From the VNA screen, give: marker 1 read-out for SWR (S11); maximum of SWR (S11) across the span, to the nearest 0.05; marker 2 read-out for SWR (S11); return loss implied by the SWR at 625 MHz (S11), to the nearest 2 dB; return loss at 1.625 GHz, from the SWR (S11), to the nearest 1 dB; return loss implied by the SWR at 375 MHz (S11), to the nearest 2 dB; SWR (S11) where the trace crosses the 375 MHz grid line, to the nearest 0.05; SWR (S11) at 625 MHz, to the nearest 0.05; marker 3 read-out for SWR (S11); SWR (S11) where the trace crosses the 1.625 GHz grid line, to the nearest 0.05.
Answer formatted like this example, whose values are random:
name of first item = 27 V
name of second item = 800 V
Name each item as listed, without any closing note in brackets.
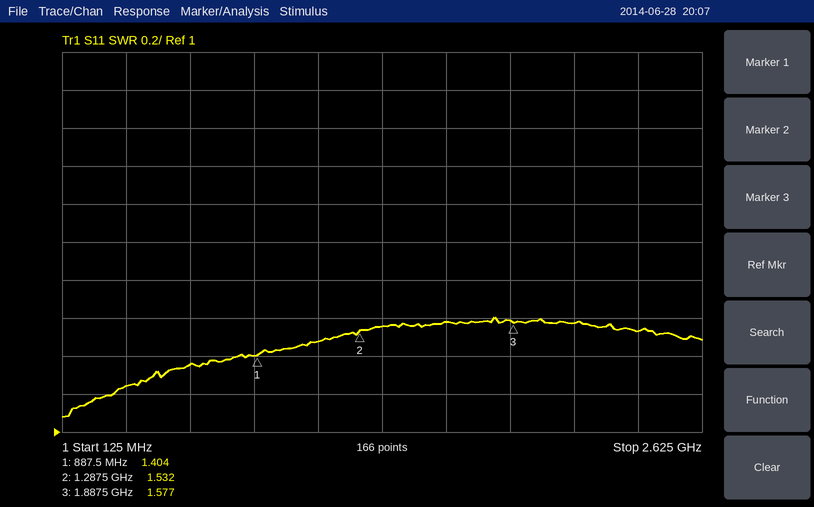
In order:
marker 1 read-out for SWR = 1.404
maximum of SWR (S11) across the span, to the nearest 0.05 = 1.60
marker 2 read-out for SWR = 1.532
return loss implied by the SWR at 625 MHz (S11), to the nearest 2 dB = 16 dB
return loss at 1.625 GHz, from the SWR (S11), to the nearest 1 dB = 13 dB
return loss implied by the SWR at 375 MHz (S11), to the nearest 2 dB = 20 dB
SWR (S11) where the trace crosses the 375 MHz grid line, to the nearest 0.05 = 1.25
SWR (S11) at 625 MHz, to the nearest 0.05 = 1.35
marker 3 read-out for SWR = 1.577
SWR (S11) where the trace crosses the 1.625 GHz grid line, to the nearest 0.05 = 1.60
